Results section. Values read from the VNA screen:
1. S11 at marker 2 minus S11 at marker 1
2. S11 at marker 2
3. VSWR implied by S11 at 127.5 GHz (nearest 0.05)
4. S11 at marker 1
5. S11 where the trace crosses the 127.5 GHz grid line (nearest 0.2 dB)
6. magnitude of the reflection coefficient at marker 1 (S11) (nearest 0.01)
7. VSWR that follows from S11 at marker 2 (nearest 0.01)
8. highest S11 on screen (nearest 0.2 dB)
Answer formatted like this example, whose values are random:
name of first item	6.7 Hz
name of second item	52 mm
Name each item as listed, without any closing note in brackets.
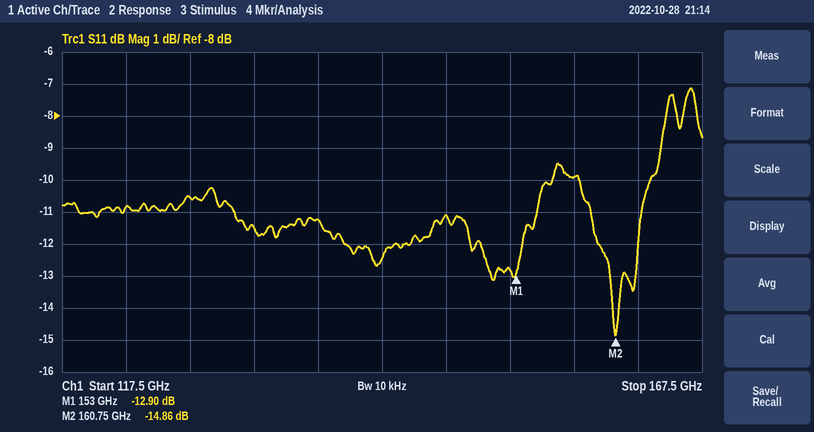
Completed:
S11 at marker 2 minus S11 at marker 1	-1.96 dB
S11 at marker 2	-14.86 dB
VSWR implied by S11 at 127.5 GHz	1.85
S11 at marker 1	-12.90 dB
S11 where the trace crosses the 127.5 GHz grid line	-10.6 dB
magnitude of the reflection coefficient at marker 1 (S11)	0.23
VSWR that follows from S11 at marker 2	1.44
highest S11 on screen	-7.2 dB
